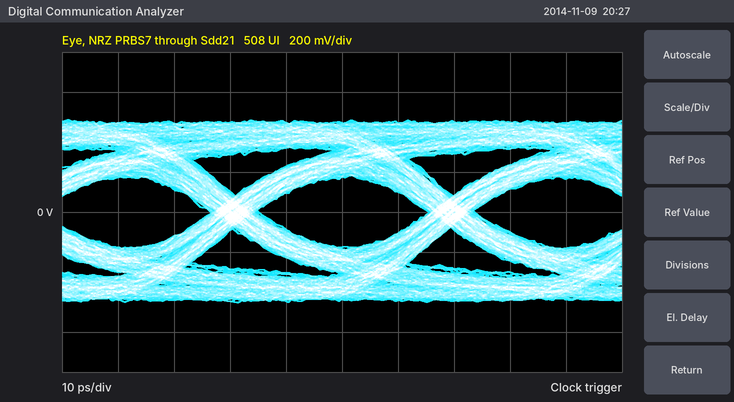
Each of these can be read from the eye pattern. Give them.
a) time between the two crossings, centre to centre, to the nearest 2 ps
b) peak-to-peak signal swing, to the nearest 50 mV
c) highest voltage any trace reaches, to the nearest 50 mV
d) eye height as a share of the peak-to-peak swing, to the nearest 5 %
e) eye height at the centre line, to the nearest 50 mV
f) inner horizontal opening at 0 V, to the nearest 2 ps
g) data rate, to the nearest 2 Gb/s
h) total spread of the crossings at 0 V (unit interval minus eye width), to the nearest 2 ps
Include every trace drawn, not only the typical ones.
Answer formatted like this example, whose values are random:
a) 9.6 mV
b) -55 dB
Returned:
a) 38 ps
b) 900 mV
c) 450 mV
d) 40 %
e) 350 mV
f) 30 ps
g) 26 Gb/s
h) 8 ps
